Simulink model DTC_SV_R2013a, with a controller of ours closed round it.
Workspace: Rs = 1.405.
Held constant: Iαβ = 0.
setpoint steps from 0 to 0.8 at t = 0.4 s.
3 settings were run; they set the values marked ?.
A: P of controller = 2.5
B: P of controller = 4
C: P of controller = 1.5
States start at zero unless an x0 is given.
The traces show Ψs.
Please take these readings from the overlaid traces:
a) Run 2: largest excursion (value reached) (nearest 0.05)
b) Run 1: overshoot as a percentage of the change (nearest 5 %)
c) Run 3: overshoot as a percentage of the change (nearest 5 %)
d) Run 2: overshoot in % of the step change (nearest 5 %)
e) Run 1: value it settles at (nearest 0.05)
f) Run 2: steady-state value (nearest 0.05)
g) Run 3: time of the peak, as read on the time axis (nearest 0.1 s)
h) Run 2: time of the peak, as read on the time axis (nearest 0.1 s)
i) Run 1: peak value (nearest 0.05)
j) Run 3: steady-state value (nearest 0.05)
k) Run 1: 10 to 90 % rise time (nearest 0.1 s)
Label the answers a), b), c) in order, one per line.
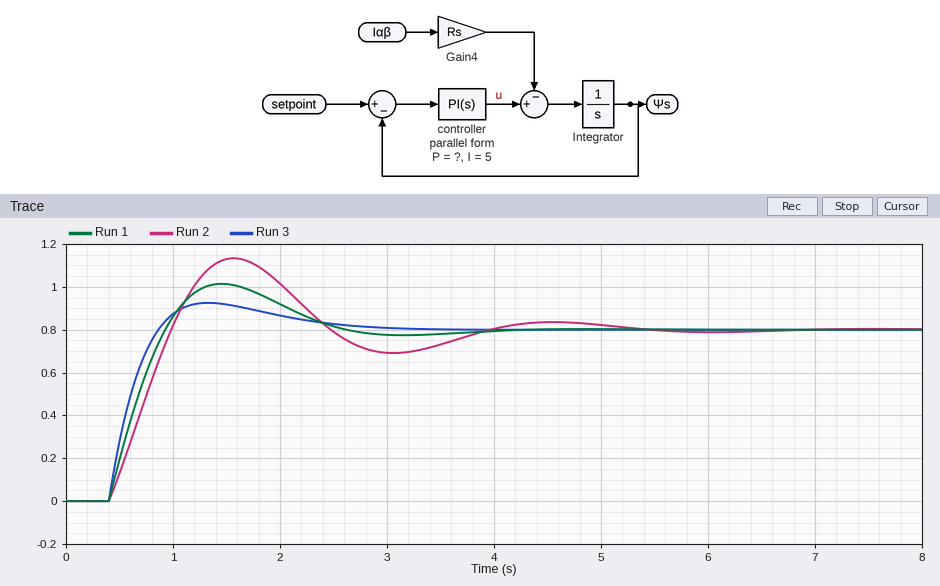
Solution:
a) 1.15
b) 25 %
c) 15 %
d) 40 %
e) 0.80
f) 0.80
g) 1.3 s
h) 1.6 s
i) 1.00
j) 0.80
k) 0.4 s
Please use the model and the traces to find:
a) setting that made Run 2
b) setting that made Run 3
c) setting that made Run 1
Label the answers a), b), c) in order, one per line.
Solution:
a) C
b) B
c) A
